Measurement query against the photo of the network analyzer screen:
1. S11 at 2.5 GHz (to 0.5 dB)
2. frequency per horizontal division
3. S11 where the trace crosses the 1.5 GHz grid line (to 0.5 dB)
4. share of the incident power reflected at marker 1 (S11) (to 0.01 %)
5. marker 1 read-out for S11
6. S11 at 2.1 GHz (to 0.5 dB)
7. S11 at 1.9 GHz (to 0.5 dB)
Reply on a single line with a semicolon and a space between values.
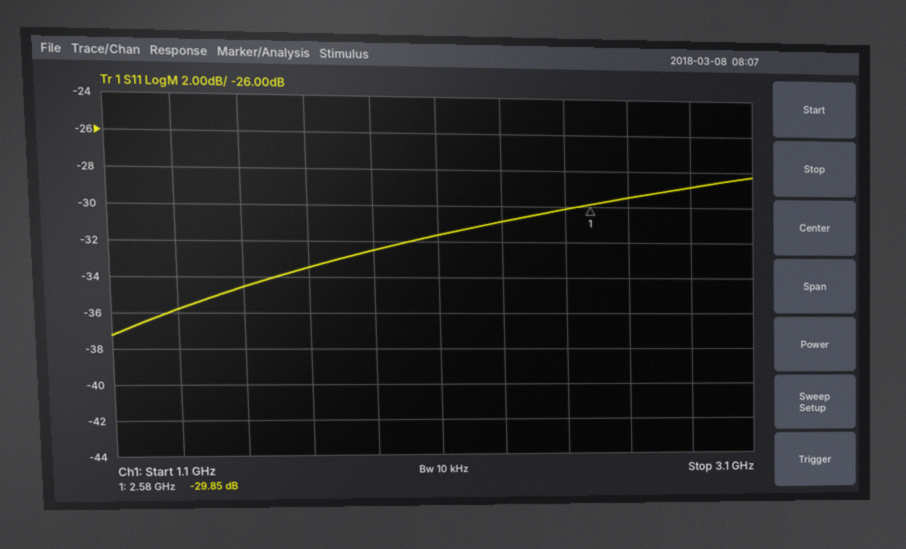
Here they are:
-30.0 dB; 200 MHz; -34.5 dB; 0.10 %; -29.85 dB; -31.5 dB; -32.5 dB
